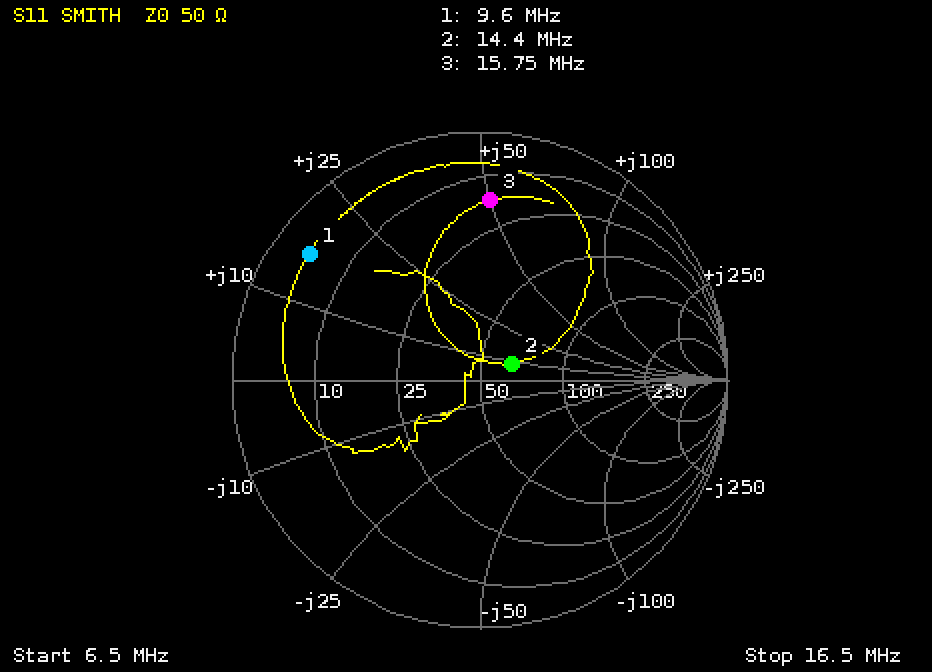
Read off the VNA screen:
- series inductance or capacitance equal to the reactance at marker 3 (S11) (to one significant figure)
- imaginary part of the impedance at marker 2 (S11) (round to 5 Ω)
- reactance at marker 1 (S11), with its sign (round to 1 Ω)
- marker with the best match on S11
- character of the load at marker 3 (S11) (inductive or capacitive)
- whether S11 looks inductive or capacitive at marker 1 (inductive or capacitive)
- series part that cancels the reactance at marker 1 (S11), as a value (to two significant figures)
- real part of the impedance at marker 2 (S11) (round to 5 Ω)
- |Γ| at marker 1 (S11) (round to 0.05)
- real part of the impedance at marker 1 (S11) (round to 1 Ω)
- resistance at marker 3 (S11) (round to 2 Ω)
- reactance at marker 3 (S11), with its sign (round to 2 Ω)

500 nH
+10 Ω
+16 Ω
marker 2
inductive
inductive
1.0 nF
65 Ω
0.85
4 Ω
16 Ω
+50 Ω
